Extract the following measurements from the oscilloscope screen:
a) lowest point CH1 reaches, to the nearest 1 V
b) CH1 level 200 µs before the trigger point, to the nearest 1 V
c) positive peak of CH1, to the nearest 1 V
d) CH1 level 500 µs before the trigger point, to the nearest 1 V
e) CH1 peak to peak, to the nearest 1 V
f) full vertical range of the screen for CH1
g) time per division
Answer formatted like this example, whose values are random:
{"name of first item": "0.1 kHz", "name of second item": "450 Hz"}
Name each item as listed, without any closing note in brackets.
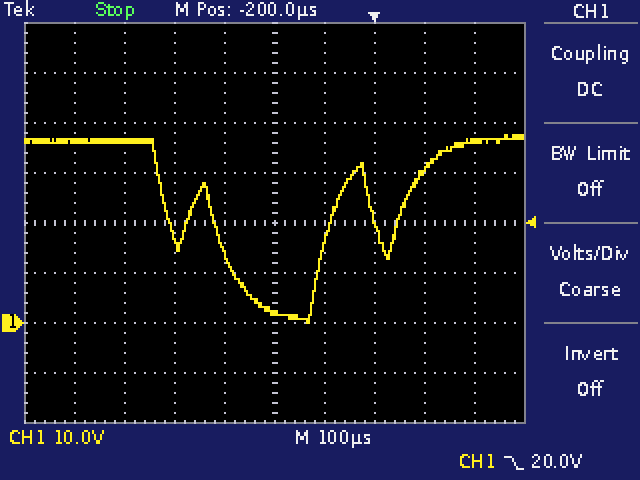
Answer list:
{"lowest point CH1 reaches, to the nearest 1 V": "0 V", "CH1 level 200 µs before the trigger point, to the nearest 1 V": "2 V", "positive peak of CH1, to the nearest 1 V": "38 V", "CH1 level 500 µs before the trigger point, to the nearest 1 V": "36 V", "CH1 peak to peak, to the nearest 1 V": "38 V", "full vertical range of the screen for CH1": "80 V", "time per division": "100 µs"}
